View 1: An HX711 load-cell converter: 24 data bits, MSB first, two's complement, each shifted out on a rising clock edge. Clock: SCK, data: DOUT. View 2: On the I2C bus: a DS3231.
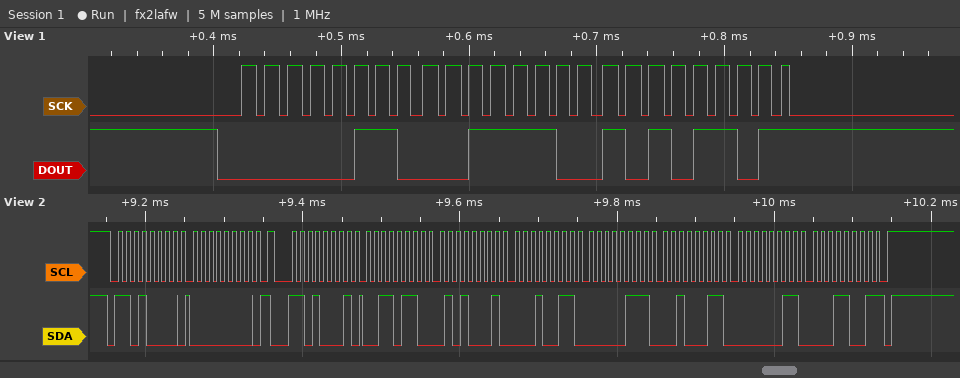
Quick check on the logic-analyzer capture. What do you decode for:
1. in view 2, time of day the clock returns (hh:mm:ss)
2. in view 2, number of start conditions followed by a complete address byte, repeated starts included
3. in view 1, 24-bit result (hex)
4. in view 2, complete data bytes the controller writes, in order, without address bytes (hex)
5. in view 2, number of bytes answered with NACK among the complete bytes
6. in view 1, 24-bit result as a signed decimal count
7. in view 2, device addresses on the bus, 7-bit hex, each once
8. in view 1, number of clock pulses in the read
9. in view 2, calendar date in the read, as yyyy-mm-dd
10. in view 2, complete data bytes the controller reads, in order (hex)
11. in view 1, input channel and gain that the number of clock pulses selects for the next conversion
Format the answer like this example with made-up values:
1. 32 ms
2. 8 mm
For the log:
1. 13:51:36
2. 2
3. 0x063CAD
4. 00
5. 1
6. 408749
7. 0x68
8. 25
9. 2019-03-23
10. 36 51 13 07 23 03 19
11. channel A, gain 128
